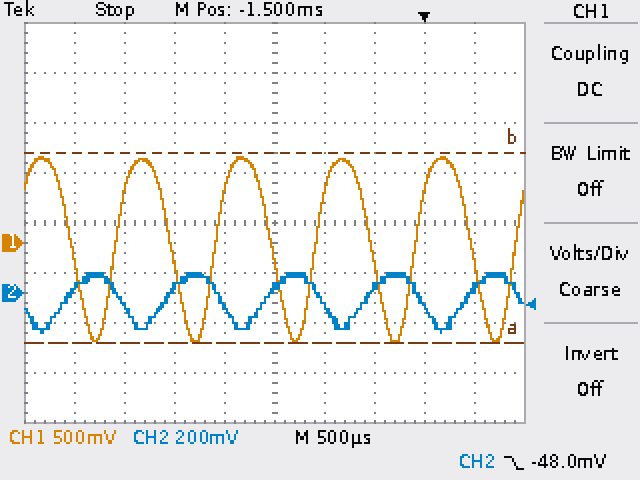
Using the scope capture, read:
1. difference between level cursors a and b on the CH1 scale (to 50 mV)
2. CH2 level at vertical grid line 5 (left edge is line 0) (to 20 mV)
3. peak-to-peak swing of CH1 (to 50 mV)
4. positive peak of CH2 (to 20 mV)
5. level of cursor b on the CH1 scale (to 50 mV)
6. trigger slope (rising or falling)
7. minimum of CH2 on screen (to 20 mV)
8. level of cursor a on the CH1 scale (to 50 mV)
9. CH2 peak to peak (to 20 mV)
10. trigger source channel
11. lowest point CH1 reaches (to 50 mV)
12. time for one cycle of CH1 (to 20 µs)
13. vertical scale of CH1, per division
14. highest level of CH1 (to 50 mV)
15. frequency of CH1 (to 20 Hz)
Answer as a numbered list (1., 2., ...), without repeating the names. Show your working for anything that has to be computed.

1. 1.90 V
2. 20 mV
3. 850 mV − (-1.00 V) = 1.85 V
4. 80 mV
5. 900 mV
6. falling
7. -160 mV
8. -1.00 V
9. 80 mV − (-160 mV) = 240 mV
10. CH2
11. -1.00 V
12. 1.00 ms
13. 500 mV
14. 850 mV
15. 1 / 1.00 ms ≈ 1.00 kHz
